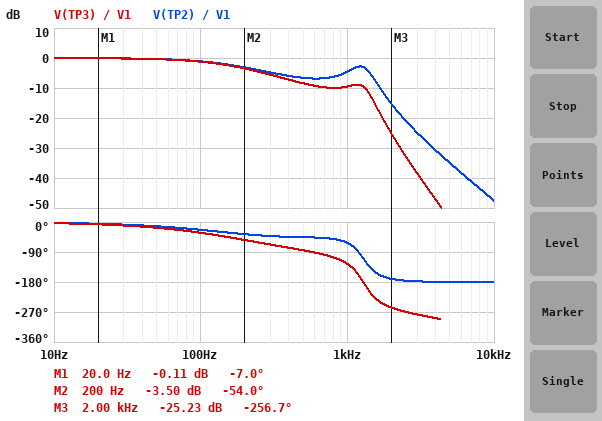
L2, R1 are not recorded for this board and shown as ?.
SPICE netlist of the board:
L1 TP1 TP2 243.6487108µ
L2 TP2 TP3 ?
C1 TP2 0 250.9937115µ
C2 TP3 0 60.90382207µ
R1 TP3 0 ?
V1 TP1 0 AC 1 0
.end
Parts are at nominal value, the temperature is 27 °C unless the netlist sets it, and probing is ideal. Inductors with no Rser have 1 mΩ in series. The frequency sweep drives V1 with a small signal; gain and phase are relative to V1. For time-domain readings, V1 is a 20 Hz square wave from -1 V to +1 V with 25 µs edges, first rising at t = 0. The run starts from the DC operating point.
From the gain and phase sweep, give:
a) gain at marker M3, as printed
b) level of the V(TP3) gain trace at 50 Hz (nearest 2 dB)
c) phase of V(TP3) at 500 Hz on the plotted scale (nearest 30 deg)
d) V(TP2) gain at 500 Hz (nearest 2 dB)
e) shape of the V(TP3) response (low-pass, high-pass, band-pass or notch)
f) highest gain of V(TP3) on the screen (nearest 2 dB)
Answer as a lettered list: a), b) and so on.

a) -25.23 dB
b) 0 dB
c) -90 deg
d) -6 dB
e) low-pass
f) 0 dB
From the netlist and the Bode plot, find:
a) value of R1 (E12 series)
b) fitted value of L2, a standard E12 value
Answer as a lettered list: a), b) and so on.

a) 0.33 Ω
b) 82 µH
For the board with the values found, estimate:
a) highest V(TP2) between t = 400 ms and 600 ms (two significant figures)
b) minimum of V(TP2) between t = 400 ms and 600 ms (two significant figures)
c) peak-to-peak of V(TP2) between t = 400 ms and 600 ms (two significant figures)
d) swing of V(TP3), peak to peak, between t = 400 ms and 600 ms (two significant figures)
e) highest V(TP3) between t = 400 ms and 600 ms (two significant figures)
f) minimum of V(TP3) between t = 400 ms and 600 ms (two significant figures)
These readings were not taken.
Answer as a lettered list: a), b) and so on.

a) 1.0 V
b) -1.0 V
c) 2.0 V
d) 2.0 V
e) 990 mV
f) -990 mV
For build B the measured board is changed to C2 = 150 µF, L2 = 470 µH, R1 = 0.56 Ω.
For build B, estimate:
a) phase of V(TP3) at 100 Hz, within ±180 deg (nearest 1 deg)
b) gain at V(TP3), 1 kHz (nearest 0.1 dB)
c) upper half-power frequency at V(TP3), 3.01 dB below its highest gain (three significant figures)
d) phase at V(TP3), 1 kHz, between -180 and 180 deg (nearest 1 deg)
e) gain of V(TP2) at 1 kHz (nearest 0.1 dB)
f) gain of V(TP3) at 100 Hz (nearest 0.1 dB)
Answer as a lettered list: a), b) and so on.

a) -40 deg
b) -13.7 dB
c) 829 Hz
d) 77 deg
e) 1.2 dB
f) -1.8 dB
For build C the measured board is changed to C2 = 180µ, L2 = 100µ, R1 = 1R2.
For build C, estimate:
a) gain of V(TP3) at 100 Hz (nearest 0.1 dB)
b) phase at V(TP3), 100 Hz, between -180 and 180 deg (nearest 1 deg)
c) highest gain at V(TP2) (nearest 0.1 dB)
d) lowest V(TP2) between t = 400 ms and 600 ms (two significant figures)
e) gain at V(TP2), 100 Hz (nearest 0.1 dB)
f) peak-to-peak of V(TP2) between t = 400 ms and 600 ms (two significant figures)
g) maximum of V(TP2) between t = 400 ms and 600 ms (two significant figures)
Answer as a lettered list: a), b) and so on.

a) 0.3 dB
b) -11 deg
c) 2.4 dB
d) -1.5 V
e) 0.2 dB
f) 3.1 V
g) 1.5 V
